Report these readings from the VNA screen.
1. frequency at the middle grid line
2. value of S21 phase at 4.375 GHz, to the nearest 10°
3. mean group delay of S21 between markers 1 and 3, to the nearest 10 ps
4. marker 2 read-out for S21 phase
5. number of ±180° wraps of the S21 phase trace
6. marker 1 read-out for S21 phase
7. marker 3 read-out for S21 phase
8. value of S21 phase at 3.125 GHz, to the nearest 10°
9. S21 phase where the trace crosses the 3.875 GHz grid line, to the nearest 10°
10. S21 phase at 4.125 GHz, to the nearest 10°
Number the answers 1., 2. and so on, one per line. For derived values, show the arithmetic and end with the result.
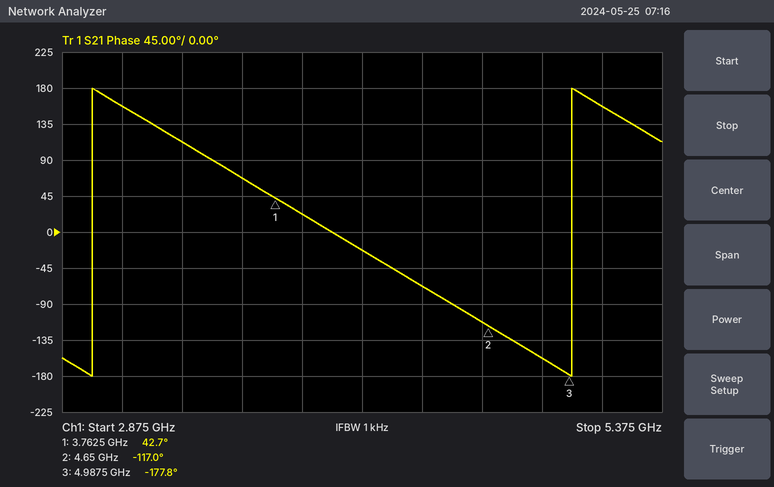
1. 4.125 GHz
2. -70°
3. −(-177.8° − (42.7°))/(360° × 1.225 GHz) ≈ 500 ps
4. -117.0°
5. 2
6. 42.7°
7. -177.8°
8. 160°
9. 20°
10. -20°
